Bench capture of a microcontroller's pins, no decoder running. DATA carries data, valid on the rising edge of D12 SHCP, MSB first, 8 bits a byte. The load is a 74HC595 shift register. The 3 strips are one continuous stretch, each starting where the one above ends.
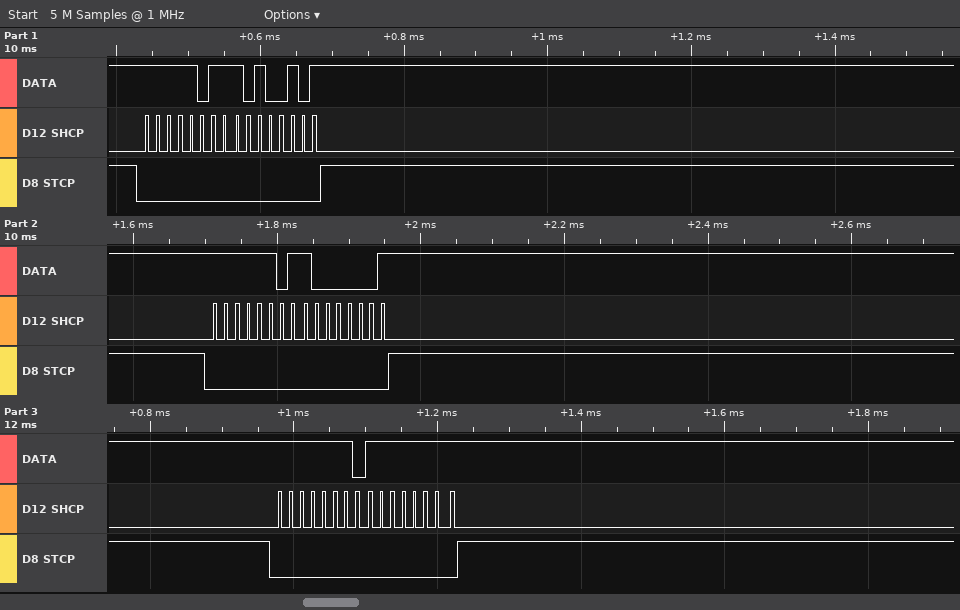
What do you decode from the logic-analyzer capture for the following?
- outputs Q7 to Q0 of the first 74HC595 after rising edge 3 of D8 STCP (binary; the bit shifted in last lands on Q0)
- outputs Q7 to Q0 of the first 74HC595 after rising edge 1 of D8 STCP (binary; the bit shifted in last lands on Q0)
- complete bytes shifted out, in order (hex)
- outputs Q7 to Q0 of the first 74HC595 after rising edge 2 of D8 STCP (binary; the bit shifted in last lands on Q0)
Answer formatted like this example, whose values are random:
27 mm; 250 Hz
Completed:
11111111; 10100101; FB A5 FD 81 FE FF; 10000001
